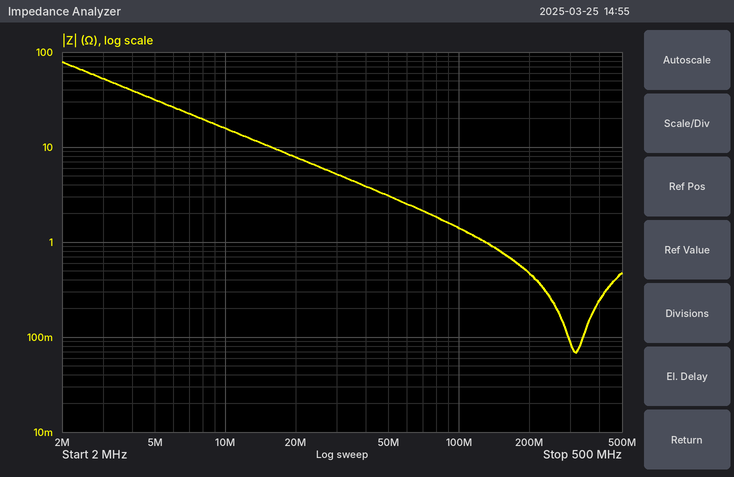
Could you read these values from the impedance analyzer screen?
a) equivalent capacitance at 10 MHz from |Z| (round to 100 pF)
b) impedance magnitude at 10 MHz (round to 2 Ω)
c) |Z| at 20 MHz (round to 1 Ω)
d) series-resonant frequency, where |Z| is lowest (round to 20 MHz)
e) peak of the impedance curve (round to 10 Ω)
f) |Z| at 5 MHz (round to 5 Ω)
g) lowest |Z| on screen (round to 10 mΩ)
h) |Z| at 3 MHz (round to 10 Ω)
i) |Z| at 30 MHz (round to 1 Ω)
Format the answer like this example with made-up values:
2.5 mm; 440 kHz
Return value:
1.0 nF; 16 Ω; 8 Ω; 320 MHz; 80 Ω; 30 Ω; 70 mΩ; 50 Ω; 5 Ω
